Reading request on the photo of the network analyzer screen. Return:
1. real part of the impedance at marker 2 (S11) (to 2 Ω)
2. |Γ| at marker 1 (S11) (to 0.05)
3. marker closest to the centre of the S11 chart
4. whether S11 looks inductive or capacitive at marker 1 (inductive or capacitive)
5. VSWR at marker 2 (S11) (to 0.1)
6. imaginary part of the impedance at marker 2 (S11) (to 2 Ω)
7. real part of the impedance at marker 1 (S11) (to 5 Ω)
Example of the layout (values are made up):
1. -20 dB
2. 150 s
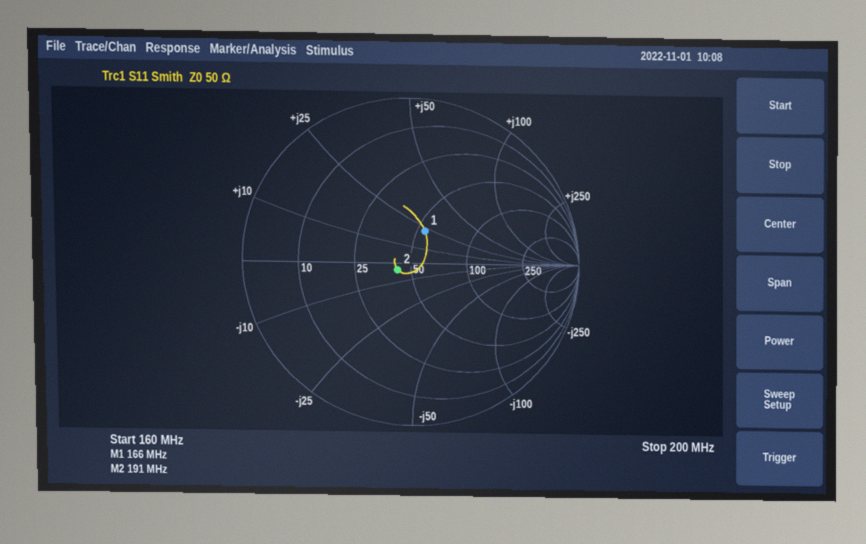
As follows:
1. 42 Ω
2. 0.20
3. marker 2
4. inductive
5. 1.2
6. -4 Ω
7. 55 Ω
